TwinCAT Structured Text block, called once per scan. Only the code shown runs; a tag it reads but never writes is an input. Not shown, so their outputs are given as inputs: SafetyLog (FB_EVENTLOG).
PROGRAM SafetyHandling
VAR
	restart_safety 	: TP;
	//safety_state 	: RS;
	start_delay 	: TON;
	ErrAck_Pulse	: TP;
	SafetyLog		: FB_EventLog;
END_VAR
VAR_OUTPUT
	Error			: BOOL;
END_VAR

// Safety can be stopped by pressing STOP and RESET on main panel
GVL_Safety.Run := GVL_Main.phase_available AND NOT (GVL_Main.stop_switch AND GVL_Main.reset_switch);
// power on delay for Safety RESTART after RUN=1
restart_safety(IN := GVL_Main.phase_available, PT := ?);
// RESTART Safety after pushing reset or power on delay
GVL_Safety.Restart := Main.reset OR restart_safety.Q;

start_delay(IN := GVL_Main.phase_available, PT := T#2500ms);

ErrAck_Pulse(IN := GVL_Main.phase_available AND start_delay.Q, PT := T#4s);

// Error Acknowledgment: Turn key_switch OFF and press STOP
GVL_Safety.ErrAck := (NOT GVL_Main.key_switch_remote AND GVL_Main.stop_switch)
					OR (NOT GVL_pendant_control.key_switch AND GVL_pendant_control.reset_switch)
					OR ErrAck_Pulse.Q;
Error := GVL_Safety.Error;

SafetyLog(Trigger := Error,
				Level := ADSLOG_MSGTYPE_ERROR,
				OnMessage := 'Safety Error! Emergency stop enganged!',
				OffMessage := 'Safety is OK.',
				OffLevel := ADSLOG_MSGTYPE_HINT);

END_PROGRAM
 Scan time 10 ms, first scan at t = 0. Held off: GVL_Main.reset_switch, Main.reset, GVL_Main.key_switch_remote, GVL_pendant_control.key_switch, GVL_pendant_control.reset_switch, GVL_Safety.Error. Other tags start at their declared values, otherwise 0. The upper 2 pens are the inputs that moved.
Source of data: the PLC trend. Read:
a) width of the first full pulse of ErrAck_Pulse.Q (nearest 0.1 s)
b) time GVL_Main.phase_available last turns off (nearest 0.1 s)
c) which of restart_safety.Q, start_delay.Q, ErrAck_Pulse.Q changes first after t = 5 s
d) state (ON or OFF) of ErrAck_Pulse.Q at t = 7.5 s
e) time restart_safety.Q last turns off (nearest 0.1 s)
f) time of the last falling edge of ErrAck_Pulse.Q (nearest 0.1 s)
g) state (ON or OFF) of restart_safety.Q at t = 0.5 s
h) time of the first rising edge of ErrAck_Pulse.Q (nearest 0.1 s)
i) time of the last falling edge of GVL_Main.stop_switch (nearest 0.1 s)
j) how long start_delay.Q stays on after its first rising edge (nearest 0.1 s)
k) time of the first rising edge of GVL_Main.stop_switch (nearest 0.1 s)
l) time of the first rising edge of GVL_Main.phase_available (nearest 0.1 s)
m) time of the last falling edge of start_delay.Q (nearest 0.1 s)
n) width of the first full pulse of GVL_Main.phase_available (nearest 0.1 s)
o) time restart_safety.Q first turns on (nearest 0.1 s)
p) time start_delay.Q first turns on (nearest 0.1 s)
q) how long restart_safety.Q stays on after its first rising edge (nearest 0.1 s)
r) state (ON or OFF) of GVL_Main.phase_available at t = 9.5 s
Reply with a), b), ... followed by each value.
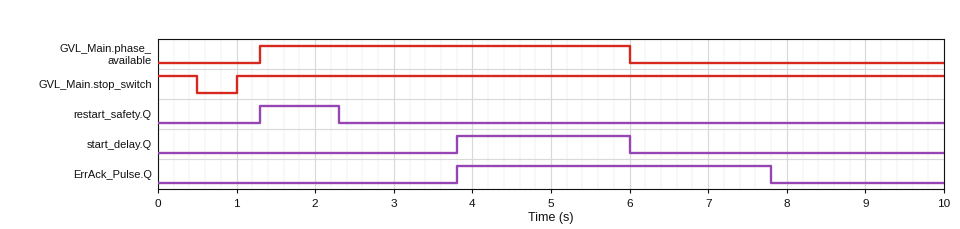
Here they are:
a) 4.0 s
b) 6.0 s
c) start_delay.Q
d) ON
e) 2.3 s
f) 7.8 s
g) OFF
h) 3.8 s
i) 0.5 s
j) 2.2 s
k) 1.0 s
l) 1.3 s
m) 6.0 s
n) 4.7 s
o) 1.3 s
p) 3.8 s
q) 1.0 s
r) OFF
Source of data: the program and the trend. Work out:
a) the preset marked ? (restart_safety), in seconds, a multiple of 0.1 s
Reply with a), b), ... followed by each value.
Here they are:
a) 1.0 s
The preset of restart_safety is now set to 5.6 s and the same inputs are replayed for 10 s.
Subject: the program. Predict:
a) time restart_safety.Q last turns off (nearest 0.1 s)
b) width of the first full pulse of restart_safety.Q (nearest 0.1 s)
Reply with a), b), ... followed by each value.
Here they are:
a) 6.9 s
b) 5.6 s
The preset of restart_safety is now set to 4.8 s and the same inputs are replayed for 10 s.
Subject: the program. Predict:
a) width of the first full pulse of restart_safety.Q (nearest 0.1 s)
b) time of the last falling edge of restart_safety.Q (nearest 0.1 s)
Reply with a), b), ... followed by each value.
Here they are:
a) 4.8 s
b) 6.1 s
